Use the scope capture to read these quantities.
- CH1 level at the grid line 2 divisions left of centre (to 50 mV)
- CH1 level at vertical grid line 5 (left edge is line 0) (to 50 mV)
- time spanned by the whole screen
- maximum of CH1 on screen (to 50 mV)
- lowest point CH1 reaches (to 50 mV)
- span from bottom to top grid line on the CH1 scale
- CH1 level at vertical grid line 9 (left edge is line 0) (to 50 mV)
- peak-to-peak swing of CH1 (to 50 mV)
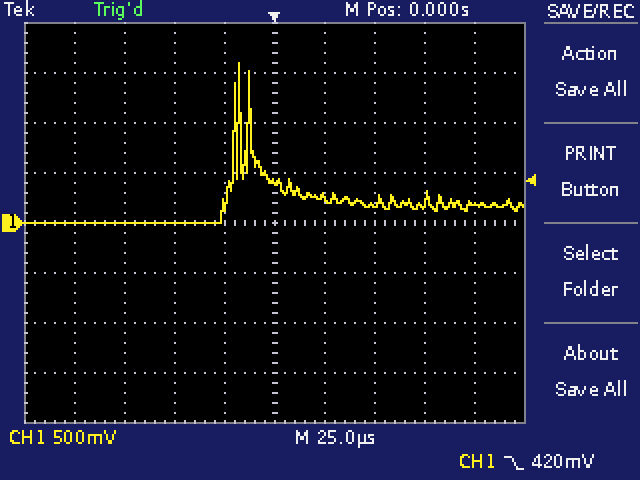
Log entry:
0 mV
400 mV
250 µs
1.60 V
0 mV
4 V
200 mV
1.60 V
